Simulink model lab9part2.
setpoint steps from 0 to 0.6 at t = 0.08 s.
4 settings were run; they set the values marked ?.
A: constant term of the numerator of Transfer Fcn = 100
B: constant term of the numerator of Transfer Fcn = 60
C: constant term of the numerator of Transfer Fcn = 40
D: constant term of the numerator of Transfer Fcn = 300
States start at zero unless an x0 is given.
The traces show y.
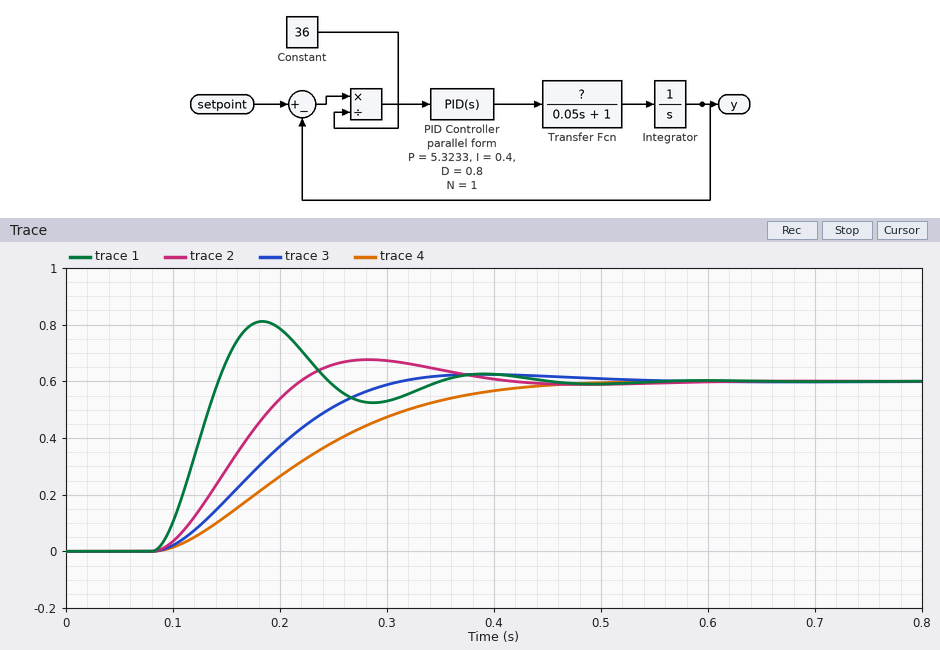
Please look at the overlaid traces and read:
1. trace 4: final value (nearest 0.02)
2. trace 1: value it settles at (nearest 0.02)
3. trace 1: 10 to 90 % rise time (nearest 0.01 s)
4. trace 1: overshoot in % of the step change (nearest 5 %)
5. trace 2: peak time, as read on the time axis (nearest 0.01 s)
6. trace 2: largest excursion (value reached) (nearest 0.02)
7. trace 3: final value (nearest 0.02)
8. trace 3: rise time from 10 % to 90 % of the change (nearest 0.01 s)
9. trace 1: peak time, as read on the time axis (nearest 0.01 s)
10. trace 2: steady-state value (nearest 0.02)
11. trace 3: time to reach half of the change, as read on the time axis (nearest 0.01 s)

0.60
0.60
0.04 s
35 %
0.28 s
0.68
0.60
0.15 s
0.18 s
0.60
0.18 s
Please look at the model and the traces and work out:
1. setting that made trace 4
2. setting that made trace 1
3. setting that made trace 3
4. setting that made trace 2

C
D
B
A
